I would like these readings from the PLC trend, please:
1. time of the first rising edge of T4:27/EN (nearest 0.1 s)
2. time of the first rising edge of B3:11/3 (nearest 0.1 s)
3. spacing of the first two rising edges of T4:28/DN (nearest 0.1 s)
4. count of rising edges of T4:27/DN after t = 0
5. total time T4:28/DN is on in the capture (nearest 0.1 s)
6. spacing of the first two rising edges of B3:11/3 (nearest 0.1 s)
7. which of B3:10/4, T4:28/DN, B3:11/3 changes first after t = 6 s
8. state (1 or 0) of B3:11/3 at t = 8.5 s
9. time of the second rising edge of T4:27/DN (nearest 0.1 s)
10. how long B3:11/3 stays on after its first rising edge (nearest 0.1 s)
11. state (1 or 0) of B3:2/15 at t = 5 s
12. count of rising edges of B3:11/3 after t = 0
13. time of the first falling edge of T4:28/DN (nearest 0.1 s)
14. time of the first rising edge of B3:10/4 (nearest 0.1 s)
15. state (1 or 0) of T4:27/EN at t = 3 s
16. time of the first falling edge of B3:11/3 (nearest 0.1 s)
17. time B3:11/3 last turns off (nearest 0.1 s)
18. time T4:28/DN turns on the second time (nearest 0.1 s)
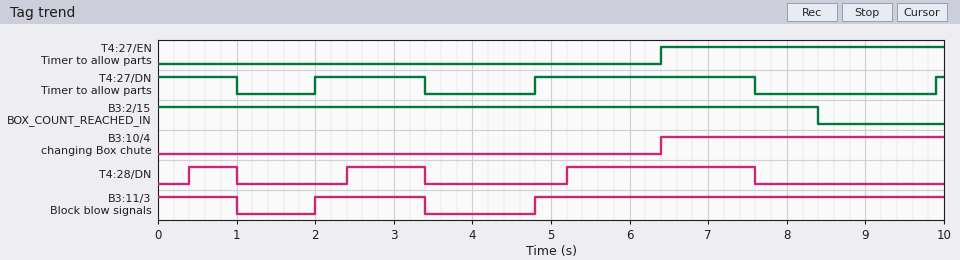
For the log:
6.4 s
2.0 s
2.0 s
3
4.0 s
2.8 s
B3:10/4
1
4.8 s
1.4 s
1
2
1.0 s
6.4 s
0
1.0 s
3.4 s
2.4 s
